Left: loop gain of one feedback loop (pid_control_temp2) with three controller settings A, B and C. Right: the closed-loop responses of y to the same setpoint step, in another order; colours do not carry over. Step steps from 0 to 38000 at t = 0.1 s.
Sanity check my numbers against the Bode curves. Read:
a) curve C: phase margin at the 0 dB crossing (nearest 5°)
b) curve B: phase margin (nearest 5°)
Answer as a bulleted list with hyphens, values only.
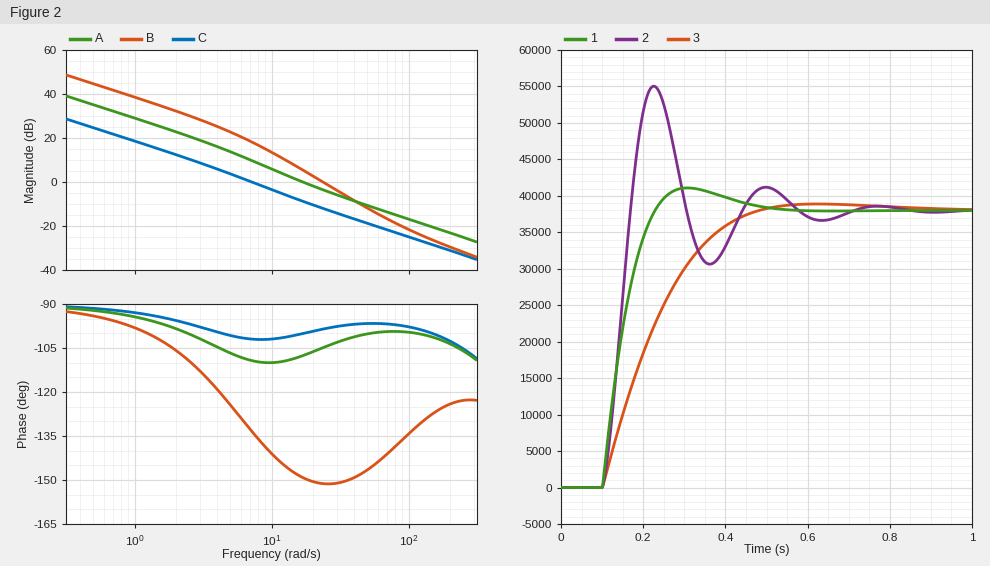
- 80°
- 30°
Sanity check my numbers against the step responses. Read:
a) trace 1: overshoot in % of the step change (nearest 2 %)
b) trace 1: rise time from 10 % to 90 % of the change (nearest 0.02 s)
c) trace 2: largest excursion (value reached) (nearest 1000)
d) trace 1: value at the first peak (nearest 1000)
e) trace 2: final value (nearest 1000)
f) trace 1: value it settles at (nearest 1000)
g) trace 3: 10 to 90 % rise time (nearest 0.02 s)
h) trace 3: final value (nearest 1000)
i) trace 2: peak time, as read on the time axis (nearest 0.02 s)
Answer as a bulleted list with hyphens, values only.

- 8 %
- 0.10 s
- 55000
- 41000
- 38000
- 38000
- 0.24 s
- 38000
- 0.22 s
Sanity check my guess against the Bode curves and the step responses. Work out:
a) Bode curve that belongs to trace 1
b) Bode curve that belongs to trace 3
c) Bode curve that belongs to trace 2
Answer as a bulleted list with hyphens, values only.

- A
- C
- B
